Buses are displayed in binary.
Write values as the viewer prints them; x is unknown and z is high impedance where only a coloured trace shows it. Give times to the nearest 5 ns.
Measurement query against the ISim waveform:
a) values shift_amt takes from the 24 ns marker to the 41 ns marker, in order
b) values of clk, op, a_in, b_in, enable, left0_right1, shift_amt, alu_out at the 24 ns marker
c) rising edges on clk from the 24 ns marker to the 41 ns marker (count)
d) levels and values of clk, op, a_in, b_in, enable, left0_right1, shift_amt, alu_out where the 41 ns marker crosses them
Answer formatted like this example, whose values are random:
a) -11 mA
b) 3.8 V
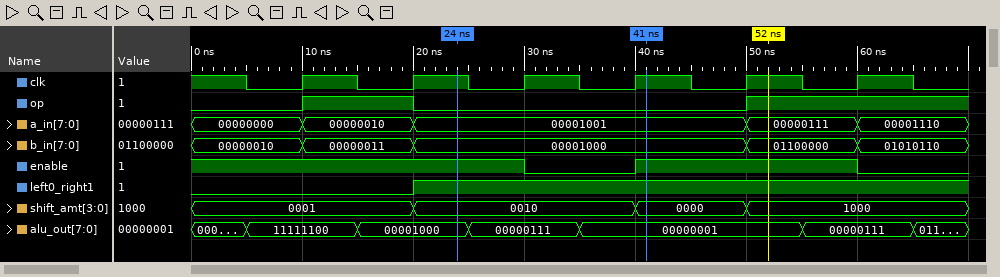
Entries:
a) 0010, 0000
b) clk=1, op=0, a_in=00001001, b_in=00001000, enable=1, left0_right1=1, shift_amt=0010, alu_out=00001000
c) 2
d) clk=1, op=0, a_in=00001001, b_in=00001000, enable=1, left0_right1=1, shift_amt=0000, alu_out=00000001
